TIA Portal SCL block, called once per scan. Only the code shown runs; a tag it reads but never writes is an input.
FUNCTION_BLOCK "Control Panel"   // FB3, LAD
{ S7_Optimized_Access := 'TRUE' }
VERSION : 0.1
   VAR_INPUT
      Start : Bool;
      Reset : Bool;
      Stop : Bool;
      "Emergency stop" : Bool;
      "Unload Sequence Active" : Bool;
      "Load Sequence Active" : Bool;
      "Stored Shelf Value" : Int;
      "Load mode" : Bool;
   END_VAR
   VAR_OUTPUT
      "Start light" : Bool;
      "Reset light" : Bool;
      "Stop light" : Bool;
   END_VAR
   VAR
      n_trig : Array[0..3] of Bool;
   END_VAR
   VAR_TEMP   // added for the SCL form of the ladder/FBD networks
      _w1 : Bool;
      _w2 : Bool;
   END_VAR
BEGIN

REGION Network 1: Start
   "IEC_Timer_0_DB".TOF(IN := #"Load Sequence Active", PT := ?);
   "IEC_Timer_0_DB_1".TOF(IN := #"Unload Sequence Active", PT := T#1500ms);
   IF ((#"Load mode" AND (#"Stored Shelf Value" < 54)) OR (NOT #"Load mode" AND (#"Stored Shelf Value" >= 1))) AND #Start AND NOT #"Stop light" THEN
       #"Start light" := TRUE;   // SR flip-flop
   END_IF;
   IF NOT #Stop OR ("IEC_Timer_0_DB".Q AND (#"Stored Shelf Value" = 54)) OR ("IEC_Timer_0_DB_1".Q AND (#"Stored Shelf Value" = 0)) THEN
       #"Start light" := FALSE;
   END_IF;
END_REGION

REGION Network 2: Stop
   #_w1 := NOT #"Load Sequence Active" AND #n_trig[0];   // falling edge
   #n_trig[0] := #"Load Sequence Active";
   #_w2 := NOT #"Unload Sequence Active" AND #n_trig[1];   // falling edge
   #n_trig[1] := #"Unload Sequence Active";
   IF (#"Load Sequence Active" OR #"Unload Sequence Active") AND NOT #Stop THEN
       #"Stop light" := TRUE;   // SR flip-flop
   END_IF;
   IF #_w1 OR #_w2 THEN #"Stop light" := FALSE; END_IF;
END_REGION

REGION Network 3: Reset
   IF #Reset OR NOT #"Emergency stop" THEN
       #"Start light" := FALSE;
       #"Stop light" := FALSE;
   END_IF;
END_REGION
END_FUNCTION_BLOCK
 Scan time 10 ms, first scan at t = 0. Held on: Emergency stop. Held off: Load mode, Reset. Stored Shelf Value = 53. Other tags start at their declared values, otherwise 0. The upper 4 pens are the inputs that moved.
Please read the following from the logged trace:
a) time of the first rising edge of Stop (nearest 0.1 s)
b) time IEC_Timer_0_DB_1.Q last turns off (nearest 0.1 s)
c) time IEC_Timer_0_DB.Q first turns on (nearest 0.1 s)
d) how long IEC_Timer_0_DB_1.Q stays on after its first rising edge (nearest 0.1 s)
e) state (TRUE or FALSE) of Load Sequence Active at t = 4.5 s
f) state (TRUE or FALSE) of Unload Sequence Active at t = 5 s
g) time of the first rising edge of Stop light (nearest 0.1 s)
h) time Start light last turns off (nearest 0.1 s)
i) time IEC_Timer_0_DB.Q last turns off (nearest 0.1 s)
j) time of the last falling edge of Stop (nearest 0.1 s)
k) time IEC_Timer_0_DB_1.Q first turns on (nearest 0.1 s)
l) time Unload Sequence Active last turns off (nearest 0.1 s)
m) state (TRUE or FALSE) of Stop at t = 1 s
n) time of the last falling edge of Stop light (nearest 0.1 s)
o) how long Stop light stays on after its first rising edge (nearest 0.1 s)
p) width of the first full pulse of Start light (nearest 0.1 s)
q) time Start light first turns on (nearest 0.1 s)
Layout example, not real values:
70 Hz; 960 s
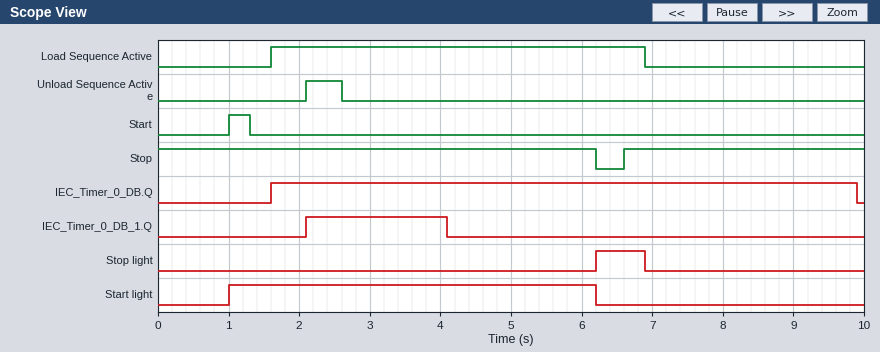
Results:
6.6 s; 4.1 s; 1.6 s; 2.0 s; TRUE; FALSE; 6.2 s; 6.2 s; 9.9 s; 6.2 s; 2.1 s; 2.6 s; TRUE; 6.9 s; 0.7 s; 5.2 s; 1.0 s
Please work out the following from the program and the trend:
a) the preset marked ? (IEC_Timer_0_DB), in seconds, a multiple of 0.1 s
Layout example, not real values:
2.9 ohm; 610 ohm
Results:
3.0 s
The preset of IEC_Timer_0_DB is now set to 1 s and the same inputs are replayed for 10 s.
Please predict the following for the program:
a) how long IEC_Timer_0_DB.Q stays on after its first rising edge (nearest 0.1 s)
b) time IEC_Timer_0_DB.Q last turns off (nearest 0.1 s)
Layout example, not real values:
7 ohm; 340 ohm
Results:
6.3 s; 7.9 s
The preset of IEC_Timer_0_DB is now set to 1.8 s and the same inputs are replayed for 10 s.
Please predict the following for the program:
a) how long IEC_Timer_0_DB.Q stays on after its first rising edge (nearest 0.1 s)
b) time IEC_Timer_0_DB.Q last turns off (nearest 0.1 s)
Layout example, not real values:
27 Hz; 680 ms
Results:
7.1 s; 8.7 s
